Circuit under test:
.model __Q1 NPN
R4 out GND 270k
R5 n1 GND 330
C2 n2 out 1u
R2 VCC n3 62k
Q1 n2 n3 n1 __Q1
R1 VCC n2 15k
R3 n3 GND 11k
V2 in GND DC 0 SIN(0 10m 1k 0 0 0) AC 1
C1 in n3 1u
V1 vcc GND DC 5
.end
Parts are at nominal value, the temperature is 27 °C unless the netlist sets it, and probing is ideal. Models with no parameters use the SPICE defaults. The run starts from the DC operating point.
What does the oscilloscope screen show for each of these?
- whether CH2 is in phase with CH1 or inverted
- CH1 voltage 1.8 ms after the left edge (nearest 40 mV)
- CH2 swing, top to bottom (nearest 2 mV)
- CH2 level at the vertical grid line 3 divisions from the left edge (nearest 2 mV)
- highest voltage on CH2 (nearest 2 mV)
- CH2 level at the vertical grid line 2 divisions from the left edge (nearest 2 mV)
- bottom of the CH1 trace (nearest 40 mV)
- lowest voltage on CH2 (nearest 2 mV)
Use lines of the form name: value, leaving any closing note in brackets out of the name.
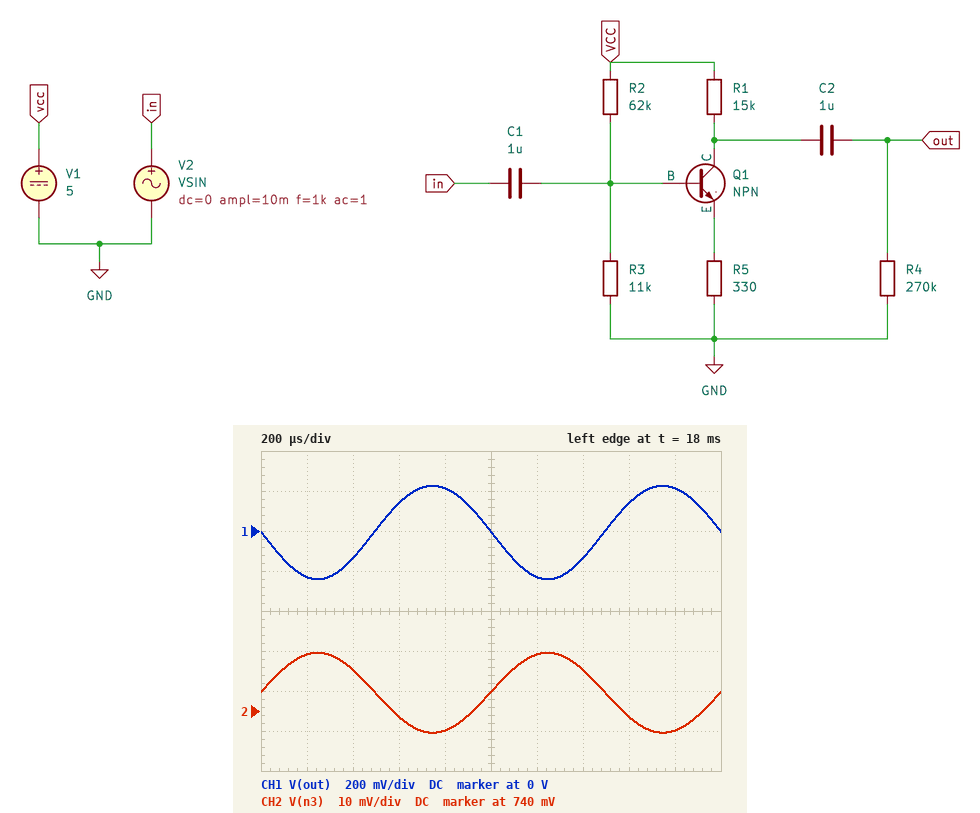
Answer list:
whether CH2 is in phase with CH1 or inverted: inverted
CH1 voltage 1.8 ms after the left edge: 200 mV
CH2 swing, top to bottom: 20 mV
CH2 level at the vertical grid line 3 divisions from the left edge: 738 mV
highest voltage on CH2: 754 mV
CH2 level at the vertical grid line 2 divisions from the left edge: 750 mV
bottom of the CH1 trace: -240 mV
lowest voltage on CH2: 734 mV
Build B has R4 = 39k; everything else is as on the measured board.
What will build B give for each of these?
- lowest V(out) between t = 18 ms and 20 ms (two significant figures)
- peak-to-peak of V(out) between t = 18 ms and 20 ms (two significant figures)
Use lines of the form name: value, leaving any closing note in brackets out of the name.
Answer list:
lowest V(out) between t = 18 ms and 20 ms: -180 mV
peak-to-peak of V(out) between t = 18 ms and 20 ms: 360 mV
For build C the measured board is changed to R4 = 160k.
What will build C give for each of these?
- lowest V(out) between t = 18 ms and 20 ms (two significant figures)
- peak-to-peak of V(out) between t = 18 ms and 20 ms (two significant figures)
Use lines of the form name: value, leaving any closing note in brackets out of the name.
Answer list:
lowest V(out) between t = 18 ms and 20 ms: -230 mV
peak-to-peak of V(out) between t = 18 ms and 20 ms: 450 mV
